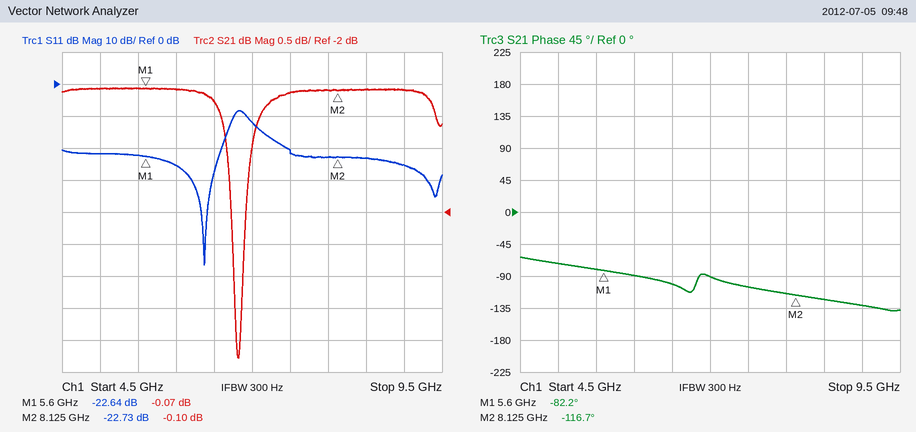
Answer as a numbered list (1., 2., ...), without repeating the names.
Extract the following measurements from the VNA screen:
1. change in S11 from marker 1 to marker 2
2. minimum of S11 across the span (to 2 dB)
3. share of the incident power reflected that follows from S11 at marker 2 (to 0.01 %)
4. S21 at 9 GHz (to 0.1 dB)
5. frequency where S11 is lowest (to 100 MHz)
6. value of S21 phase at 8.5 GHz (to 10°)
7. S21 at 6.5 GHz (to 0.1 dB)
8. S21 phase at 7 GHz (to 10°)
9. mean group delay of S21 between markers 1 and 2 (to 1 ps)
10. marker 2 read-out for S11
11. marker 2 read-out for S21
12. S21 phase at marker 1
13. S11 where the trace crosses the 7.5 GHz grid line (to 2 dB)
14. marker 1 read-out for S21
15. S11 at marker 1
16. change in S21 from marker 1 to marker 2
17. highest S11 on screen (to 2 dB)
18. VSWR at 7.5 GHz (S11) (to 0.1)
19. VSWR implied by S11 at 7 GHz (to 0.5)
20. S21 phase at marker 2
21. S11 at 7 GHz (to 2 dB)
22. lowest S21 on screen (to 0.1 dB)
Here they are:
1. -0.09 dB
2. -56 dB
3. 0.53 %
4. -0.1 dB
5. 6.4 GHz
6. -120°
7. -0.3 dB
8. -90°
9. 38 ps
10. -22.73 dB
11. -0.10 dB
12. -82.2°
13. -20 dB
14. -0.07 dB
15. -22.64 dB
16. -0.03 dB
17. -8 dB
18. 1.2
19. 1.5
20. -116.7°
21. -12 dB
22. -4.3 dB
